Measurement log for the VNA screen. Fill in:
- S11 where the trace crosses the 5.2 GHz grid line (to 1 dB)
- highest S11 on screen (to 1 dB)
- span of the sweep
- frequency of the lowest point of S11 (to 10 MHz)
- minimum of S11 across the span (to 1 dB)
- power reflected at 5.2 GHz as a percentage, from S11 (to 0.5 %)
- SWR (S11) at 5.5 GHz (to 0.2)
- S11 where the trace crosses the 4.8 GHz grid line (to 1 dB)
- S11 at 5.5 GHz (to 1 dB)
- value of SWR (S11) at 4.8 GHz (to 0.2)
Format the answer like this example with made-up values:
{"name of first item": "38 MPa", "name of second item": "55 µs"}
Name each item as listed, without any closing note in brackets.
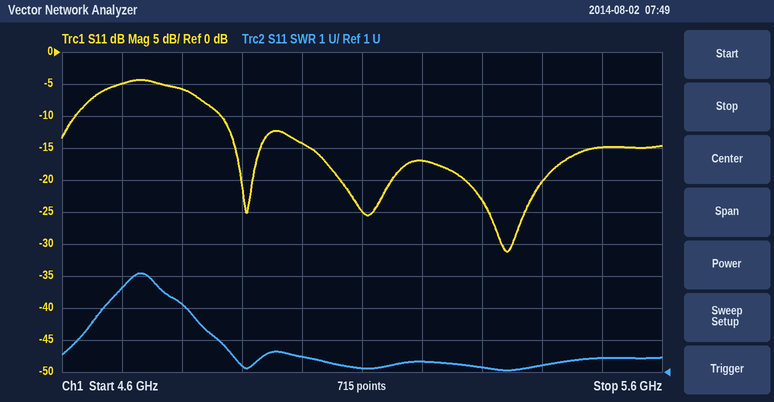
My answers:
{"S11 where the trace crosses the 5.2 GHz grid line": "-17 dB", "highest S11 on screen": "-4 dB", "span of the sweep": "1 GHz", "frequency of the lowest point of S11": "5.34 GHz", "minimum of S11 across the span": "-31 dB", "power reflected at 5.2 GHz as a percentage, from S11": "2.0 %", "SWR (S11) at 5.5 GHz": "1.4", "S11 where the trace crosses the 4.8 GHz grid line": "-6 dB", "S11 at 5.5 GHz": "-15 dB", "value of SWR (S11) at 4.8 GHz": "3.2"}
